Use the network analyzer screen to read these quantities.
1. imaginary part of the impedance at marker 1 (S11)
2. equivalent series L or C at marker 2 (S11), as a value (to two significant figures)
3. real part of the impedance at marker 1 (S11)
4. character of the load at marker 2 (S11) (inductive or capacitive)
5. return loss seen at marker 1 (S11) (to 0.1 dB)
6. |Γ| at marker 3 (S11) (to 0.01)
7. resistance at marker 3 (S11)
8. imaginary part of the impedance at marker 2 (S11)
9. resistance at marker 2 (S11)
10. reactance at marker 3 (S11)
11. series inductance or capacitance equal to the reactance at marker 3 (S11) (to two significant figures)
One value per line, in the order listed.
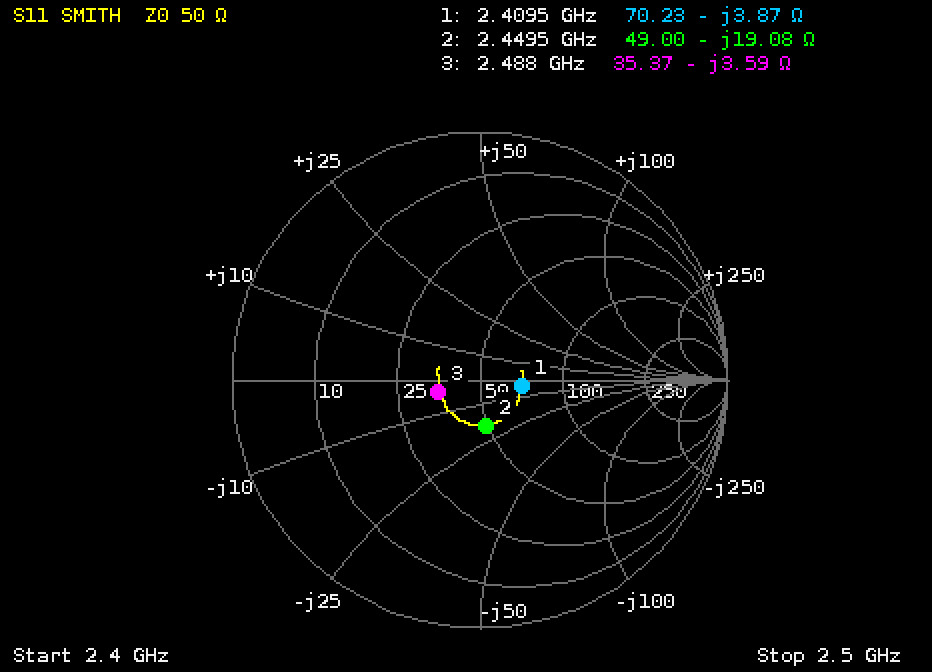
-3.87 Ω
3.4 pF
70.23 Ω
capacitive
15.3 dB
0.18
35.37 Ω
-19.08 Ω
49.00 Ω
-3.59 Ω
18 pF
